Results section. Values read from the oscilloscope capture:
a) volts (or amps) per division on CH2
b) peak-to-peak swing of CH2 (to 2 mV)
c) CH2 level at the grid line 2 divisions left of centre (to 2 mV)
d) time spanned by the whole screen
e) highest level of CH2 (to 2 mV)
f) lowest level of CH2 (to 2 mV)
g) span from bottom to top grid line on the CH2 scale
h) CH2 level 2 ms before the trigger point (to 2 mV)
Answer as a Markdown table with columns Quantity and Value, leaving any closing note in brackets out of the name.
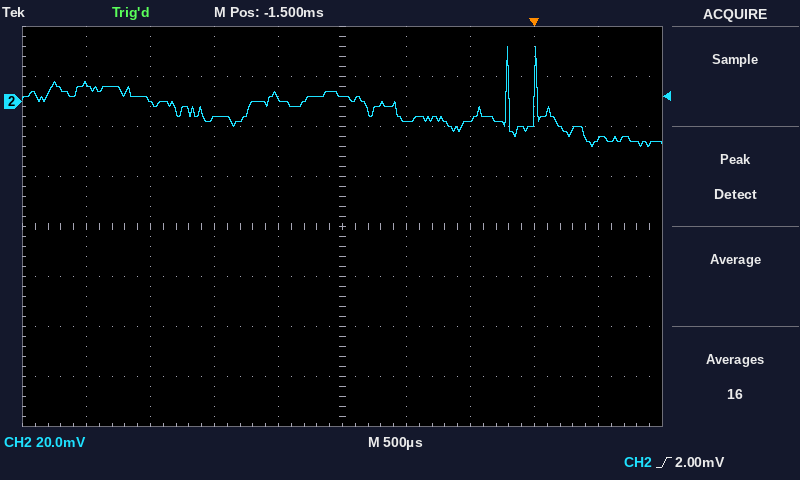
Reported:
| Quantity | Value |
|---|---|
| volts (or amps) per division on CH2 | 20 mV |
| peak-to-peak swing of CH2 | 40 mV |
| CH2 level at the grid line 2 divisions left of centre | -6 mV |
| time spanned by the whole screen | 5 ms |
| highest level of CH2 | 22 mV |
| lowest level of CH2 | -18 mV |
| span from bottom to top grid line on the CH2 scale | 160 mV |
| CH2 level 2 ms before the trigger point | 2 mV |
